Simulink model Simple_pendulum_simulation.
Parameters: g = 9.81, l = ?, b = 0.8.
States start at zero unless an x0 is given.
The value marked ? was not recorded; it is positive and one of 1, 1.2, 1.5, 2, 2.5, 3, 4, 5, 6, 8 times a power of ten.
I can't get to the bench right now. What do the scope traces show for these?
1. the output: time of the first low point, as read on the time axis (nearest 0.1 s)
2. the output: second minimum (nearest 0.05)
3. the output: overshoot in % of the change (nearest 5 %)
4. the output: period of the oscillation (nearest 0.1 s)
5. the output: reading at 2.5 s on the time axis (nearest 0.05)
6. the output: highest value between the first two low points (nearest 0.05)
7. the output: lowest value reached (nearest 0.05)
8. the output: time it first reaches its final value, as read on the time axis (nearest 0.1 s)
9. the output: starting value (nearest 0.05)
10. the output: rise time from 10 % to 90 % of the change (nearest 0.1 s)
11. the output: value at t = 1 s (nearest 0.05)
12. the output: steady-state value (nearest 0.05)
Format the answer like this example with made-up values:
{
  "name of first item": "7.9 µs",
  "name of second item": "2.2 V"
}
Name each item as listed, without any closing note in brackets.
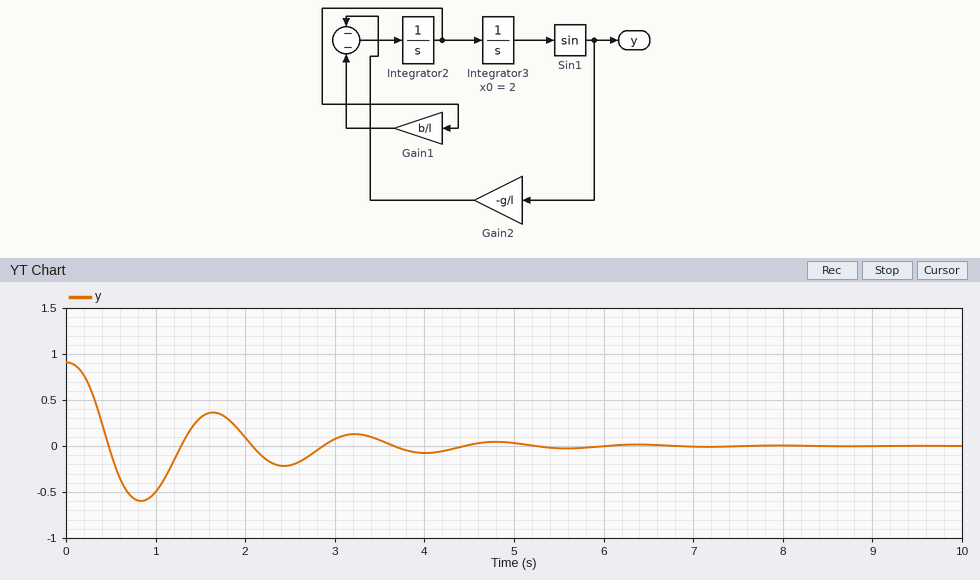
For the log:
{
  "the output: time of the first low point, as read on the time axis": "0.8 s",
  "the output: second minimum": "-0.20",
  "the output: overshoot in % of the change": "65 %",
  "the output: period of the oscillation": "1.6 s",
  "the output: reading at 2.5 s on the time axis": "-0.20",
  "the output: highest value between the first two low points": "0.35",
  "the output: lowest value reached": "-0.60",
  "the output: time it first reaches its final value, as read on the time axis": "0.5 s",
  "the output: starting value": "0.90",
  "the output: rise time from 10 % to 90 % of the change": "0.3 s",
  "the output: value at t = 1 s": "-0.50",
  "the output: steady-state value": "0.00"
}
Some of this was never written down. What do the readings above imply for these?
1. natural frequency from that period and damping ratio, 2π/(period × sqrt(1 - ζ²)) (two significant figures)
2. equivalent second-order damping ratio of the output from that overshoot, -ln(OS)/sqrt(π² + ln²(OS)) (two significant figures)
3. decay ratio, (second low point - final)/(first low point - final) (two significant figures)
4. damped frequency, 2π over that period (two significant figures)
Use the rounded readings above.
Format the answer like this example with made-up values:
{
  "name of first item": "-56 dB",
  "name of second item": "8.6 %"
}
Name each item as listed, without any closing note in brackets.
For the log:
{
  "natural frequency from that period and damping ratio, 2π/(period × sqrt(1 - ζ²))": "4.0 rad/s",
  "equivalent second-order damping ratio of the output from that overshoot, -ln(OS)/sqrt(π² + ln²(OS))": "0.14",
  "decay ratio, (second low point - final)/(first low point - final)": "0.33",
  "damped frequency, 2π over that period": "3.9 rad/s"
}
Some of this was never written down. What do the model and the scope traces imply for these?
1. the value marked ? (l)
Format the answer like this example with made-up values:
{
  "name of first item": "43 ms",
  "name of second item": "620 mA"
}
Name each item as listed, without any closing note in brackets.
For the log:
{
  "the value marked ?": "0.6"
}
